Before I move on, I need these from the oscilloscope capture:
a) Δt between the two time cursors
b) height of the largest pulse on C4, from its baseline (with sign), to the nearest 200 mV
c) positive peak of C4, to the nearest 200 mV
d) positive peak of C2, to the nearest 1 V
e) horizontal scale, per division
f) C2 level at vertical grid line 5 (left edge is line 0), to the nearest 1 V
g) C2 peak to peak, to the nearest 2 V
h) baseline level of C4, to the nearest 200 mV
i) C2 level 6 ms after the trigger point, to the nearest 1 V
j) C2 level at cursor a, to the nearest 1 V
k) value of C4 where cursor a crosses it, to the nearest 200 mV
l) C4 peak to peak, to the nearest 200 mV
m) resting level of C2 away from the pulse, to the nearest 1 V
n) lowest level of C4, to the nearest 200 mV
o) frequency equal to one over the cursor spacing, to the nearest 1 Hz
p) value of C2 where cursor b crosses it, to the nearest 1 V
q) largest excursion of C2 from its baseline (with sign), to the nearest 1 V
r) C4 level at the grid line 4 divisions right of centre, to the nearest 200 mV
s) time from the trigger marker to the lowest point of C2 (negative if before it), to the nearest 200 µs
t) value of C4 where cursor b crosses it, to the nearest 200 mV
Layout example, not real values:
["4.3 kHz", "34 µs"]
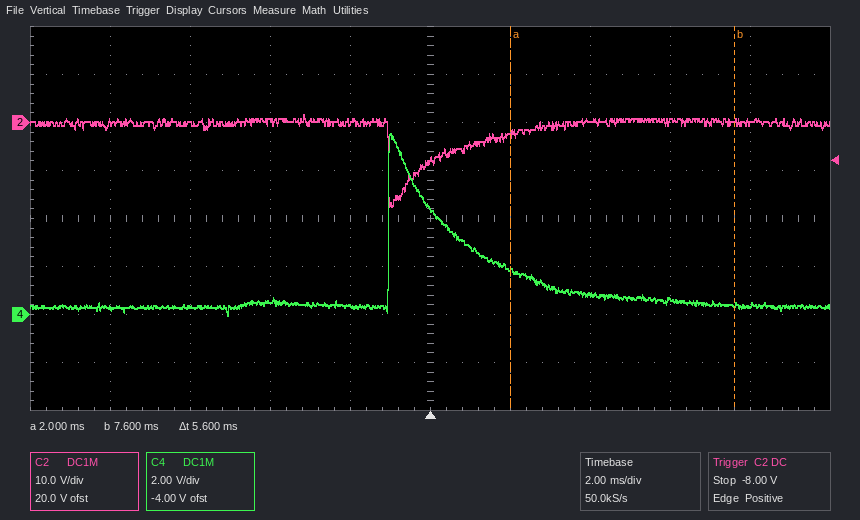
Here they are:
["5.6 ms", "+7.2 V", "7.6 V", "2 V", "2 ms", "-8 V", "20 V", "400 mV", "0 V", "-2 V", "1.8 V", "7.6 V", "0 V", "0.0 V", "179 Hz", "0 V", "-18 V", "400 mV", "-1.0 ms", "400 mV"]
